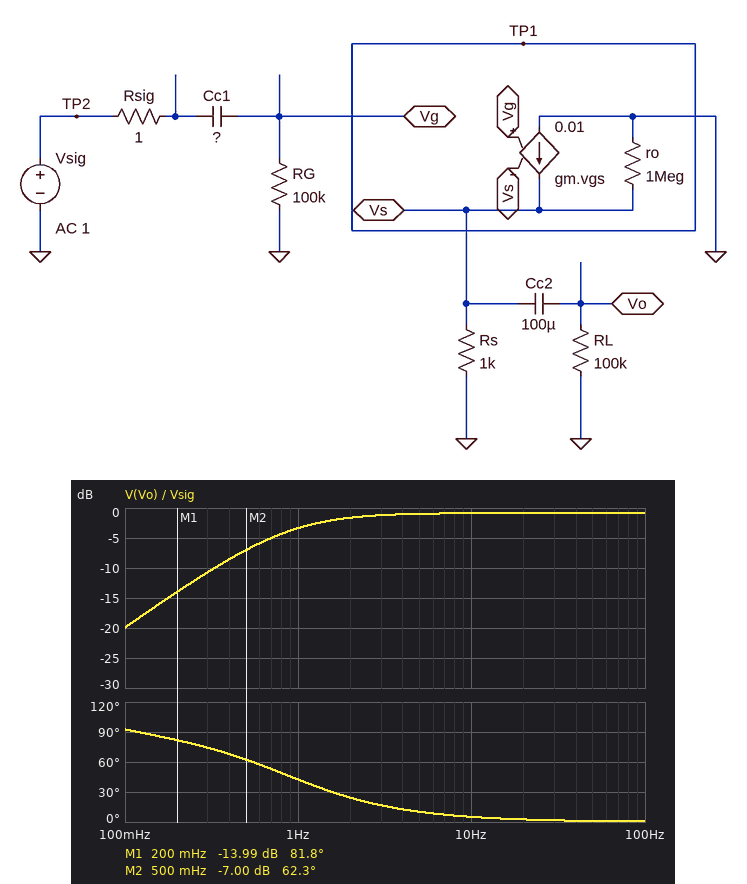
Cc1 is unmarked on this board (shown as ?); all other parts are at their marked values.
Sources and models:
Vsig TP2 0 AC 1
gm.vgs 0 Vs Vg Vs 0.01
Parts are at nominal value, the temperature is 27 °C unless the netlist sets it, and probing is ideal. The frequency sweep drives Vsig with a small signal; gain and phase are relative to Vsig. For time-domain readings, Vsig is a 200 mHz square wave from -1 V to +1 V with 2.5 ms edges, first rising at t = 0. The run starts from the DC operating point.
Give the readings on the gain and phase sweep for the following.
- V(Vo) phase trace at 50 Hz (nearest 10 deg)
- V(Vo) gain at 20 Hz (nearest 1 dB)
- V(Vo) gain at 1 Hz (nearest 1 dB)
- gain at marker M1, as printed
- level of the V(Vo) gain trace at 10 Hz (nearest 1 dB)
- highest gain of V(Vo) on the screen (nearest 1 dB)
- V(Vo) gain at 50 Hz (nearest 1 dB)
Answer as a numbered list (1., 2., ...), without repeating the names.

1. 0 deg
2. -1 dB
3. -3 dB
4. -13.99 dB
5. -1 dB
6. -1 dB
7. -1 dB
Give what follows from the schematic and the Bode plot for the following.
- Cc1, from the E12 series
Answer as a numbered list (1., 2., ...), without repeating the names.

1. 1.8 µF
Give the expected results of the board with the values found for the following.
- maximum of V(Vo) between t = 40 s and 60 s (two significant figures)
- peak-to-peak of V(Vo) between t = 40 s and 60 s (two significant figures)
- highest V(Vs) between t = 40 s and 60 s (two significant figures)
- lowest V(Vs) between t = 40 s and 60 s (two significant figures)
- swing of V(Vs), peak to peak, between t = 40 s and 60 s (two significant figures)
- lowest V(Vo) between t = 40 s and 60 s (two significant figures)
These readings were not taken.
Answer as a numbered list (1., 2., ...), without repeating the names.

1. 1.8 V
2. 3.6 V
3. 1.8 V
4. -1.8 V
5. 3.6 V
6. -1.8 V
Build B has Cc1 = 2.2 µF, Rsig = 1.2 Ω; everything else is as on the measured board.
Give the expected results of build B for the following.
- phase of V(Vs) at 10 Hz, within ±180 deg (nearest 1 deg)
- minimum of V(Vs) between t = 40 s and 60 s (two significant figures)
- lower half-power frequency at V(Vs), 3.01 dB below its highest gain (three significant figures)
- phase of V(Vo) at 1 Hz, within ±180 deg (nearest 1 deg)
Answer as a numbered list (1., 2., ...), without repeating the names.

1. 4 deg
2. -1.8 V
3. 723 mHz
4. 37 deg
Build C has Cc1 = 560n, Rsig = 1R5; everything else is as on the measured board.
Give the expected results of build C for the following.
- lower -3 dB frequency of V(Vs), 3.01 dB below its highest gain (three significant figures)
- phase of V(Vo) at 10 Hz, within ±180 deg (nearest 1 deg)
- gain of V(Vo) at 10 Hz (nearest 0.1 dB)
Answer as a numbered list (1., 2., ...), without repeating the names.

1. 2.84 Hz
2. 16 deg
3. -1.2 dB
